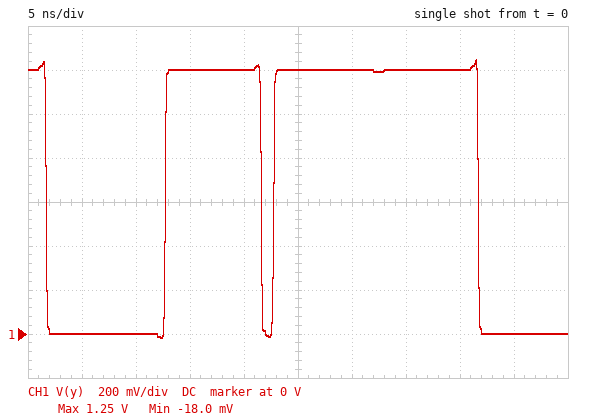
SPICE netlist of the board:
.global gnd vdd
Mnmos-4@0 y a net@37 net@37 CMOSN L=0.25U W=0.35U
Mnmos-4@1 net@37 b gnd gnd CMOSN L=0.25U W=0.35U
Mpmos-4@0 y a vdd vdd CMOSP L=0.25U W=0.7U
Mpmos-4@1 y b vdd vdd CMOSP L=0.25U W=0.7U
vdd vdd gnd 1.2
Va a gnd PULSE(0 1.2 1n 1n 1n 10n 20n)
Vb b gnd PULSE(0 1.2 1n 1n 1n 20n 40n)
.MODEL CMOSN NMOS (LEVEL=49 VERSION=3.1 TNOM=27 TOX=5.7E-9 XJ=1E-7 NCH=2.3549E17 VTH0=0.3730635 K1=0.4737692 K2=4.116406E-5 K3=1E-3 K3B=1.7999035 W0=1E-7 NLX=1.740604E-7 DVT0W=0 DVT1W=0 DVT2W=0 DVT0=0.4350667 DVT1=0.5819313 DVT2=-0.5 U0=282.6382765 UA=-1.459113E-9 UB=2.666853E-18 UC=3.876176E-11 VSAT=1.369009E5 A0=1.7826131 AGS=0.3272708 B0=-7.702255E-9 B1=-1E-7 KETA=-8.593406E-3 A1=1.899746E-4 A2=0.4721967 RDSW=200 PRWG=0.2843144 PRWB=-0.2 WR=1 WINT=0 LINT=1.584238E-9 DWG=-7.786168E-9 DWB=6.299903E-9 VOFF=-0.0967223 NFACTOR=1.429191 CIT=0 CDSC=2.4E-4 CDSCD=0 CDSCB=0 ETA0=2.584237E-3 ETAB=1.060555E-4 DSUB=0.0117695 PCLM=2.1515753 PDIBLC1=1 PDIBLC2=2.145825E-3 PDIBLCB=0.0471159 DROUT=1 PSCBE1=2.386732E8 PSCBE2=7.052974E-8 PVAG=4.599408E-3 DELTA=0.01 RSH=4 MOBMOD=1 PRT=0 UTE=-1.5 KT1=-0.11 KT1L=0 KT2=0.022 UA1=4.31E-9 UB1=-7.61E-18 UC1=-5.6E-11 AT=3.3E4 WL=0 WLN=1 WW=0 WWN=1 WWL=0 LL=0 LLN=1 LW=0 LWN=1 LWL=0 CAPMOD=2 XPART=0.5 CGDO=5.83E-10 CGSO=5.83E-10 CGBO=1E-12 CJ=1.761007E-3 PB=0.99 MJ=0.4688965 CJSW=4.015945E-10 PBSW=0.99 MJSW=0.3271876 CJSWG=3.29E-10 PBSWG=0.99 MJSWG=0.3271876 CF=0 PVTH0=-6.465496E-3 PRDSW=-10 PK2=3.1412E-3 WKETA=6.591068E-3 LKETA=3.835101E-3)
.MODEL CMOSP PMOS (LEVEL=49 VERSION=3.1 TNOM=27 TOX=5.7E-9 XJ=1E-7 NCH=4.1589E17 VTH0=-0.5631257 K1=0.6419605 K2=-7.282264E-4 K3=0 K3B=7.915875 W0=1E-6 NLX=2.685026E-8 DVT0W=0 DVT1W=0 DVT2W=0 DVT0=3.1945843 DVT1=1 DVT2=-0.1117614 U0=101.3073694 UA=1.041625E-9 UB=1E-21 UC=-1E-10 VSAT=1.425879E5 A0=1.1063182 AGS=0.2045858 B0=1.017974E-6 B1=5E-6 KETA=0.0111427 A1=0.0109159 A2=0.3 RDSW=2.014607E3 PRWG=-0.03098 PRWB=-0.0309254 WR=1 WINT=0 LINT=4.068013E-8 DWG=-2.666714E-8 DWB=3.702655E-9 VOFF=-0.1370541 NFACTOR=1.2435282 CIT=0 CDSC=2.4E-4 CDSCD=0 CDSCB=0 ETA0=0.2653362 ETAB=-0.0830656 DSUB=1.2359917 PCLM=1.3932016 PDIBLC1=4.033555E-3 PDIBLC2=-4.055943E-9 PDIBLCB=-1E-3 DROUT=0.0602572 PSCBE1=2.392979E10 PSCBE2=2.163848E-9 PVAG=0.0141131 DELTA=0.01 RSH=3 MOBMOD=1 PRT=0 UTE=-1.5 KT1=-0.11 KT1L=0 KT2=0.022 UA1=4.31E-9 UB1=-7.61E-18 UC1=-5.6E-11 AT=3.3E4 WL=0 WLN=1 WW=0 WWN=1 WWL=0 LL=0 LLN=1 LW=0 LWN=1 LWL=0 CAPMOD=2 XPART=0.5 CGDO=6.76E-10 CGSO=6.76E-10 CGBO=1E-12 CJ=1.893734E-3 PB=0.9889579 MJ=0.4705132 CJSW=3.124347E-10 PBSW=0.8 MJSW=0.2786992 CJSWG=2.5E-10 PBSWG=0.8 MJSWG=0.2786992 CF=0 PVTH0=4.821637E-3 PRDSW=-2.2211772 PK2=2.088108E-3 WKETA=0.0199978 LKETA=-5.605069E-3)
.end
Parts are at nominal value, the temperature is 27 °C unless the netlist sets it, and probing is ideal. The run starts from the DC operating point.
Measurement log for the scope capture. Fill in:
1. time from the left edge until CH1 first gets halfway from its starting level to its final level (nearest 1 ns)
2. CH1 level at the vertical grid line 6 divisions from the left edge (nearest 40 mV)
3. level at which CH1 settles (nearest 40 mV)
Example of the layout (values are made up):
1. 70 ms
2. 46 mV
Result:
1. 2 ns
2. 1.20 V
3. 0 V
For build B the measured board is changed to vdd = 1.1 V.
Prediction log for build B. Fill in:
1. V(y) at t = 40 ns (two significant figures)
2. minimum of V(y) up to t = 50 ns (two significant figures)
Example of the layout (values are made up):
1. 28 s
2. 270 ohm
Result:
1. 1.1 V
2. -24 mV
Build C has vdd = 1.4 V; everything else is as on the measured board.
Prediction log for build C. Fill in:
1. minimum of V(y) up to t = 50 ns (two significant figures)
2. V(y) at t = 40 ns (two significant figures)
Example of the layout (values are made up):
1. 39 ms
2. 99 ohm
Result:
1. -14 mV
2. 1.4 V
